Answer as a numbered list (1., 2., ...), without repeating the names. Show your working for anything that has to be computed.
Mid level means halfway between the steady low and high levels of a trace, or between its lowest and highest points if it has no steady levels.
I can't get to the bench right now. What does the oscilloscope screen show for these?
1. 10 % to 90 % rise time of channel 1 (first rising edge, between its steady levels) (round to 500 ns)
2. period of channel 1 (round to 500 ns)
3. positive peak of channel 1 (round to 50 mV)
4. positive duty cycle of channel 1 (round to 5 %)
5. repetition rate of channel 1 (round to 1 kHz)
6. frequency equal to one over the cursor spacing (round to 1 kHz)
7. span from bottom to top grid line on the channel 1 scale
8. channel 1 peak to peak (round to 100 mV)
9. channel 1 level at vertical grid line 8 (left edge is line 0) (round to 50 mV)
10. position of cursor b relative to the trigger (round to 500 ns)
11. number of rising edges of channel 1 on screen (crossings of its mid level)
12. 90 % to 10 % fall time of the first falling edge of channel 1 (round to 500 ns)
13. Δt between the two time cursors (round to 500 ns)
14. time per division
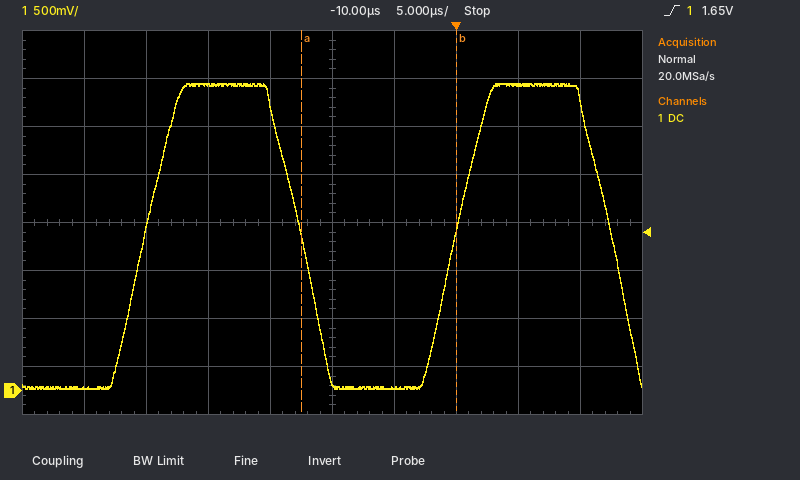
1. 4.5 µs
2. 25.0 µs
3. 3.20 V
4. 50 %
5. 1 / 25.0 µs ≈ 40 kHz
6. 1 / 12.5 µs ≈ 80 kHz
7. 4 V
8. 3.20 V
9. 3.20 V
10. 0.0 µs
11. 2
12. 4.5 µs
13. 12.5 µs
14. 5 µs
